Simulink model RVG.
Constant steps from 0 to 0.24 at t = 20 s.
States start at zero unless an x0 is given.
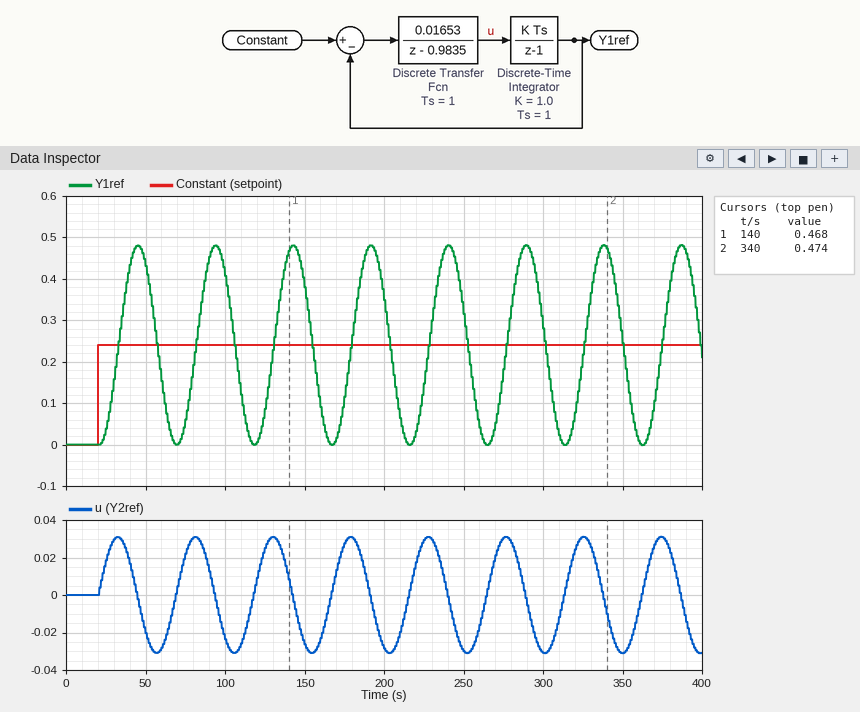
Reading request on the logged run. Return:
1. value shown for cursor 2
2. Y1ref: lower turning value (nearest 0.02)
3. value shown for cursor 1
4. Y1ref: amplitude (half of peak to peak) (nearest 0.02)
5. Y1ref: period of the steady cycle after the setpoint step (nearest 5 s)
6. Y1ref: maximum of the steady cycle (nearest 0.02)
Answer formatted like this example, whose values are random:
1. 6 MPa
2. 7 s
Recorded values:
1. 0.474
2. 0.00
3. 0.468
4. 0.24
5. 50 s
6. 0.48
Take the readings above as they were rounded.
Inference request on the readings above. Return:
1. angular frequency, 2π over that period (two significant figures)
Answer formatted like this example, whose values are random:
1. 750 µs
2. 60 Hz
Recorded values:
1. 0.13 rad/s
